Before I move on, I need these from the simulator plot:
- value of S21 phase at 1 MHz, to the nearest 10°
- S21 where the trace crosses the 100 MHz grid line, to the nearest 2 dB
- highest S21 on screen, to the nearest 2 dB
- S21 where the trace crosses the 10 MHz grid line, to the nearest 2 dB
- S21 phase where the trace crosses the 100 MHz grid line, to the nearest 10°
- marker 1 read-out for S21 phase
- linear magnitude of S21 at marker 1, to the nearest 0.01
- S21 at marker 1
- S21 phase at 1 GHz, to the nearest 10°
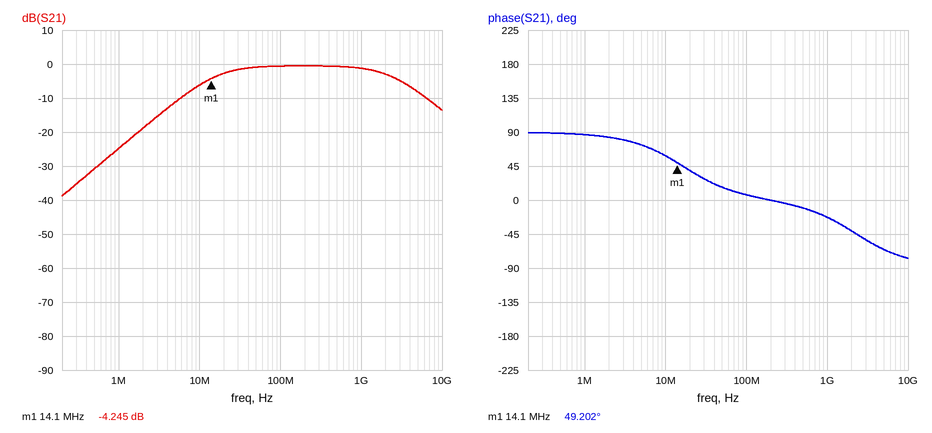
90°
0 dB
0 dB
-6 dB
10°
49.202°
0.61
-4.245 dB
-20°
